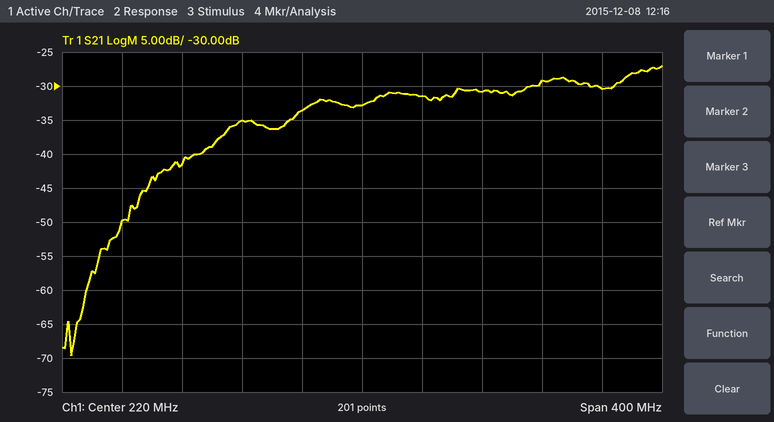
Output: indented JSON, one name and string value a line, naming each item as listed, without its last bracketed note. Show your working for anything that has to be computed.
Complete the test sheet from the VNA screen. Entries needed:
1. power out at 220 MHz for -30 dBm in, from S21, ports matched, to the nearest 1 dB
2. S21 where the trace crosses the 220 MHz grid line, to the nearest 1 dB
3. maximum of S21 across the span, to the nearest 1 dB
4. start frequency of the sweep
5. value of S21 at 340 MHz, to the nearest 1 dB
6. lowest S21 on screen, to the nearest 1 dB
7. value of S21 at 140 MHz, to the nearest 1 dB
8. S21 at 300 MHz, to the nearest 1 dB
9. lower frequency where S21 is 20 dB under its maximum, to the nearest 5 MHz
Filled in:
{
  "power out at 220 MHz for -30 dBm in, from S21, ports matched, to the nearest 1 dB": "-30 dBm + (-33 dB) = -63 dBm",
  "S21 where the trace crosses the 220 MHz grid line, to the nearest 1 dB": "-33 dB",
  "maximum of S21 across the span, to the nearest 1 dB": "-27 dB",
  "start frequency of the sweep": "20 MHz",
  "value of S21 at 340 MHz, to the nearest 1 dB": "-29 dB",
  "lowest S21 on screen, to the nearest 1 dB": "-70 dB",
  "value of S21 at 140 MHz, to the nearest 1 dB": "-35 dB",
  "S21 at 300 MHz, to the nearest 1 dB": "-31 dB",
  "lower frequency where S21 is 20 dB under its maximum, to the nearest 5 MHz": "70 MHz"
}
